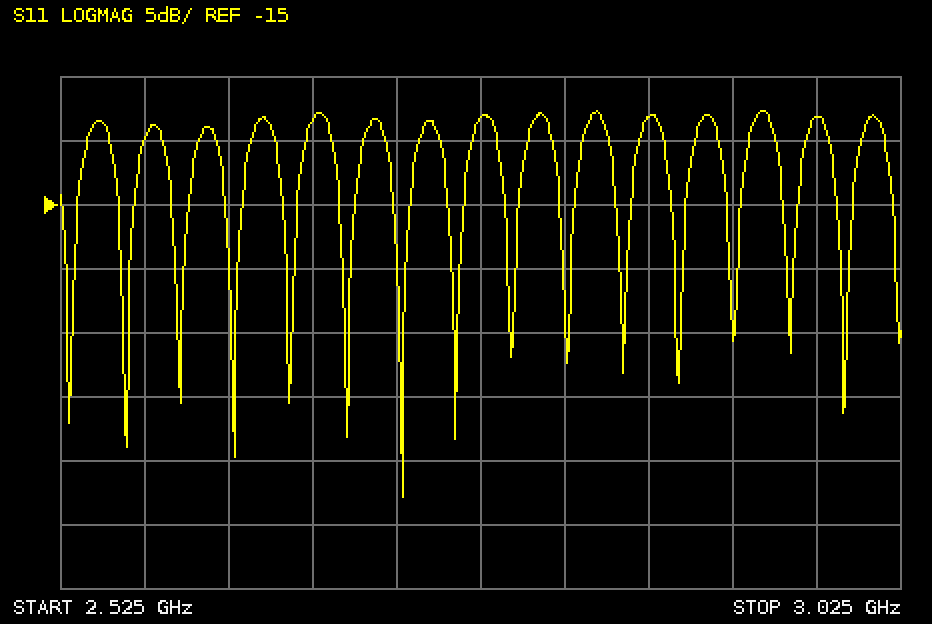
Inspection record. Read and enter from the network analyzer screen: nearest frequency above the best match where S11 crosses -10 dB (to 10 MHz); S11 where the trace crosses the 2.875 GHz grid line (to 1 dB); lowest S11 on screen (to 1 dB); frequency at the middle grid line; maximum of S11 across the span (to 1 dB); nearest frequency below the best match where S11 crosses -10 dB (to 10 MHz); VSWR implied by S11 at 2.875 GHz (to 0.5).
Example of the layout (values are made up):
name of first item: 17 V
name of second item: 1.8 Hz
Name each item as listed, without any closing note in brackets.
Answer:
nearest frequency above the best match where S11 crosses -10 dB: 2.74 GHz
S11 where the trace crosses the 2.875 GHz grid line: -8 dB
lowest S11 on screen: -38 dB
frequency at the middle grid line: 2.775 GHz
maximum of S11 across the span: -8 dB
nearest frequency below the best match where S11 crosses -10 dB: 2.72 GHz
VSWR implied by S11 at 2.875 GHz: 2.5
